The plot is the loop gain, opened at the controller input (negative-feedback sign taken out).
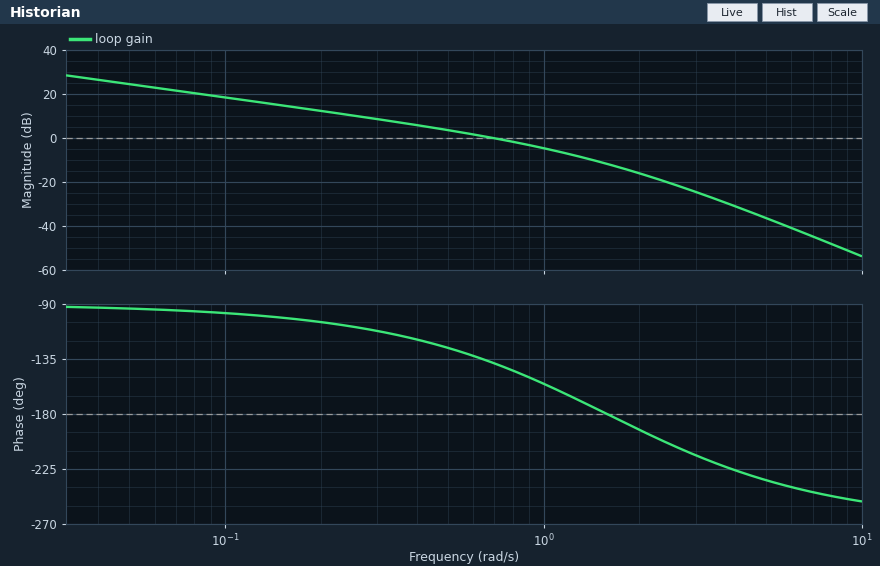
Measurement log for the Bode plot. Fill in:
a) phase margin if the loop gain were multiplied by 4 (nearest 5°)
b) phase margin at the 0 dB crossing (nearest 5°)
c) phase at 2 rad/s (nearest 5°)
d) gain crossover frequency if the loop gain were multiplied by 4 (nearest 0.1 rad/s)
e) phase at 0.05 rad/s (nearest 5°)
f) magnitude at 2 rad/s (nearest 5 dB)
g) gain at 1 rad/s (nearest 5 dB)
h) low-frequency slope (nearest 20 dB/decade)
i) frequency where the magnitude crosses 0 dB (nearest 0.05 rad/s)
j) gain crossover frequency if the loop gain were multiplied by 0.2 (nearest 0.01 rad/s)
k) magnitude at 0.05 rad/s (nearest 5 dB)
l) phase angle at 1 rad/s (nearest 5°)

0°
40°
-195°
1.6 rad/s
-95°
-15 dB
-5 dB
-20 dB/decade
0.70 rad/s
0.17 rad/s
25 dB
-155°
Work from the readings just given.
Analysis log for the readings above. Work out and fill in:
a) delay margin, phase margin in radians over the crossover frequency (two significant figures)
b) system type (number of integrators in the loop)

1.00 s
1
